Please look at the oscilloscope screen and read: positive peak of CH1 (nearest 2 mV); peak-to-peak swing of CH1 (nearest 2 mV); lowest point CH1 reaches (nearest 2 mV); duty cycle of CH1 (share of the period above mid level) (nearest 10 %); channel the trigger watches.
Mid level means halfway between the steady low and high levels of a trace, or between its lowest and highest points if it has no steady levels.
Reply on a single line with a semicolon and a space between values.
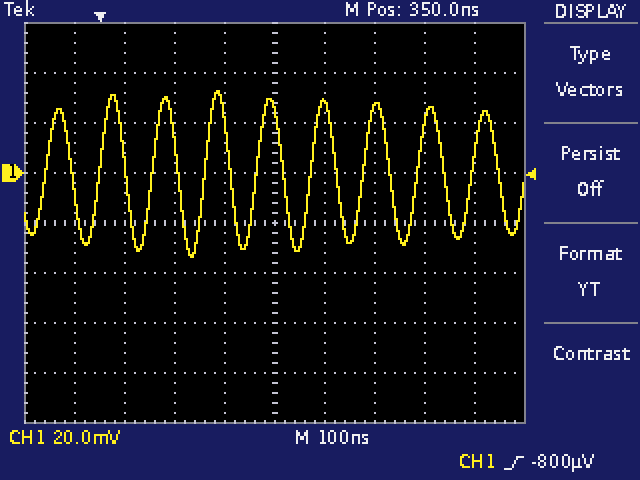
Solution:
32 mV; 66 mV; -34 mV; 50 %; CH1
